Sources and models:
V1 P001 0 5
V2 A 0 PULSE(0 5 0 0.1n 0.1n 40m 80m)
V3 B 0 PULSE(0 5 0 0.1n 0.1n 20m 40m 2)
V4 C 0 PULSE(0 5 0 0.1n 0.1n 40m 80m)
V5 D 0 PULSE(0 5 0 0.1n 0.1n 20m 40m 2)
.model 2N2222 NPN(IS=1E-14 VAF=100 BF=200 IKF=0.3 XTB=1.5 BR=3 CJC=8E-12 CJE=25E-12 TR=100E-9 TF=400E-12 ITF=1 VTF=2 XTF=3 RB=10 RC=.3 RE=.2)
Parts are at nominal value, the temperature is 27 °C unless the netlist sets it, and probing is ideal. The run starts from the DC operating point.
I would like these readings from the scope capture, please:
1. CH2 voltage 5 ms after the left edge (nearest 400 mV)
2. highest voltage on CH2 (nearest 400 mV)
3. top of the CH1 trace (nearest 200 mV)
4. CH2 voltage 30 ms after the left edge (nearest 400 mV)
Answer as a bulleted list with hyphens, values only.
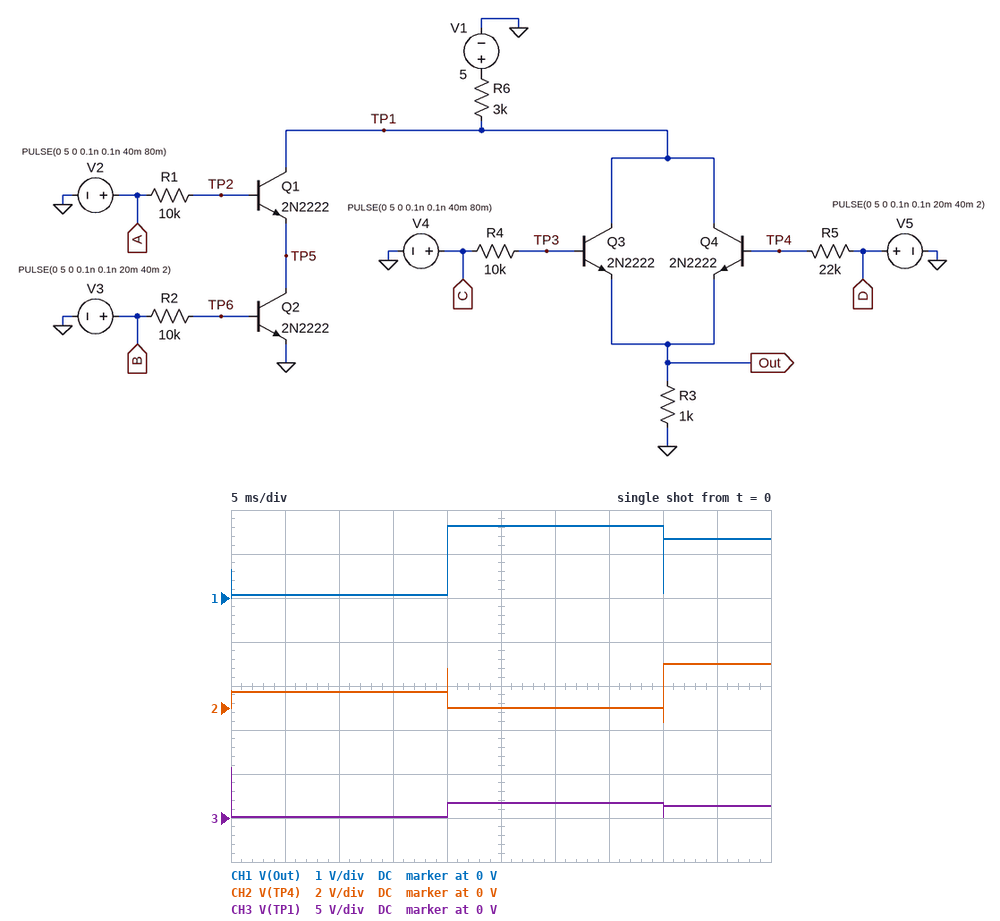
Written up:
- 800 mV
- 2.0 V
- 1.6 V
- 0 V
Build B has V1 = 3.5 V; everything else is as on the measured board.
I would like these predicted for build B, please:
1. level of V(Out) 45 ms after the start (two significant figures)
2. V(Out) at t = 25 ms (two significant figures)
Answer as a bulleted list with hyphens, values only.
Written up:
- 980 mV
- 1.3 V
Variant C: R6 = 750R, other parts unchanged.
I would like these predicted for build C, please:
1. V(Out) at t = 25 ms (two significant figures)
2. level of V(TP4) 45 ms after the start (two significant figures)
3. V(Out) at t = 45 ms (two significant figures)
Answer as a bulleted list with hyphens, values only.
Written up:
- 2.9 V
- 3.5 V
- 2.8 V
